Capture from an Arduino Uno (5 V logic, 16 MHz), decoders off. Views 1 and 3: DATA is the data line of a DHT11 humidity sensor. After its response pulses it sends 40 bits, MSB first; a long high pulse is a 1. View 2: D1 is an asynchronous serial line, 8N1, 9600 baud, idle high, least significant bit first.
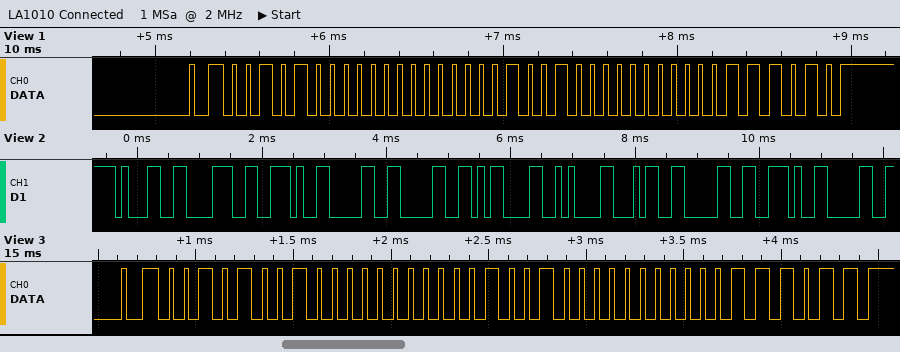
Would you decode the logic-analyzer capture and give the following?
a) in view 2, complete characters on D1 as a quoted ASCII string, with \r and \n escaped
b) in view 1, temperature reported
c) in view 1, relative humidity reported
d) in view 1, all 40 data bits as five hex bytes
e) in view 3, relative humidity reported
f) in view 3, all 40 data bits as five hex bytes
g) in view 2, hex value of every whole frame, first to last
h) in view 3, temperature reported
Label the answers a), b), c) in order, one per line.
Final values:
a) "18.00\r\n40.0"
b) 18.0 °C
c) 40 %
d) 28 00 12 00 3A
e) 41 %
f) 29 00 12 00 3B
g) 31 38 2E 30 30 0D 0A 34 30 2E 30
h) 18.0 °C
